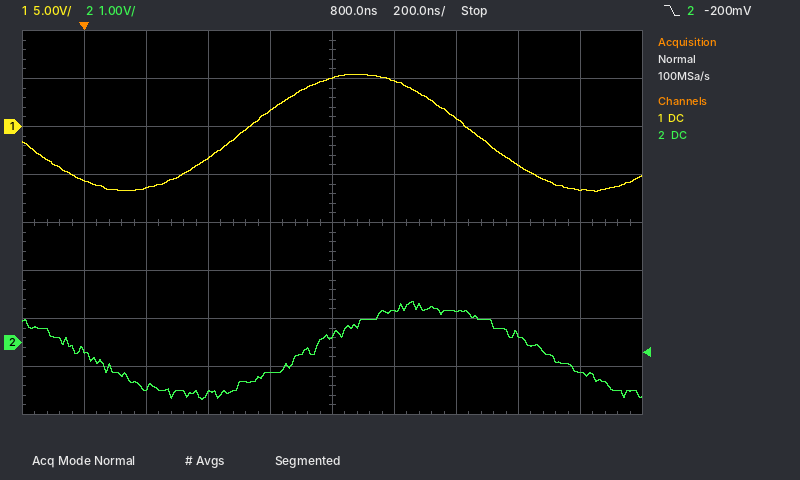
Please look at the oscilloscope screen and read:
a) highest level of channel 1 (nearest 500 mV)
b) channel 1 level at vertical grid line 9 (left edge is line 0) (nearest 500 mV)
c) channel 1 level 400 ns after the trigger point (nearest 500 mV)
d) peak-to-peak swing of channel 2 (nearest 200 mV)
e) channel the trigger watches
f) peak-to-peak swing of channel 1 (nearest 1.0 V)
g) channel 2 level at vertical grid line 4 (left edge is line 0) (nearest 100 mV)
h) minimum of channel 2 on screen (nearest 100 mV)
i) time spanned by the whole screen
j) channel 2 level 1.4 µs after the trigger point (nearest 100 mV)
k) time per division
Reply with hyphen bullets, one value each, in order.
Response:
- 5.5 V
- -6.5 V
- -3.5 V
- 2.0 V
- channel 2
- 12.0 V
- -600 mV
- -1.2 V
- 2 µs
- 200 mV
- 200 ns
